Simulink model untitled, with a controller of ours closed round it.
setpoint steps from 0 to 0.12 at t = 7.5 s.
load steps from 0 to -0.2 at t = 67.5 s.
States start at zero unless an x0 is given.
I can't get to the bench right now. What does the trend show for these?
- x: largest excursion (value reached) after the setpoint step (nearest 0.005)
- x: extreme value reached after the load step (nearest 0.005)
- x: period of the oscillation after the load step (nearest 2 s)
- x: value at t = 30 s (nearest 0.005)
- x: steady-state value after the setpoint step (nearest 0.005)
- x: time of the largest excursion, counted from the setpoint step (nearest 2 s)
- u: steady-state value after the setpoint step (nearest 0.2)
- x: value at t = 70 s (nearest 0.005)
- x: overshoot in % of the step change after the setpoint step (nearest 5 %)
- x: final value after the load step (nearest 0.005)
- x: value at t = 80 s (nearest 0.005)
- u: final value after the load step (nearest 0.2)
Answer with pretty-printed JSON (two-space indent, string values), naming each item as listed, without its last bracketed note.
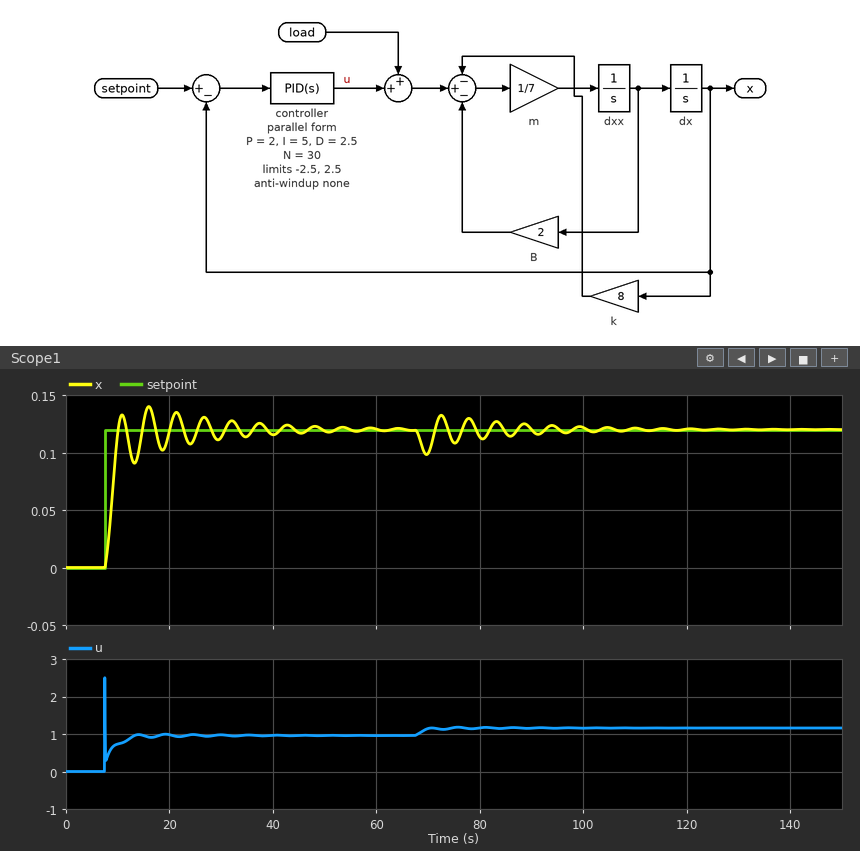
{
  "x: largest excursion (value reached) after the setpoint step": "0.140",
  "x: extreme value reached after the load step": "0.100",
  "x: period of the oscillation after the load step": "6 s",
  "x: value at t = 30 s": "0.115",
  "x: steady-state value after the setpoint step": "0.120",
  "x: time of the largest excursion, counted from the setpoint step": "8 s",
  "u: steady-state value after the setpoint step": "1.0",
  "x: value at t = 70 s": "0.100",
  "x: overshoot in % of the step change after the setpoint step": "15 %",
  "x: final value after the load step": "0.120",
  "x: value at t = 80 s": "0.115",
  "u: final value after the load step": "1.2"
}
